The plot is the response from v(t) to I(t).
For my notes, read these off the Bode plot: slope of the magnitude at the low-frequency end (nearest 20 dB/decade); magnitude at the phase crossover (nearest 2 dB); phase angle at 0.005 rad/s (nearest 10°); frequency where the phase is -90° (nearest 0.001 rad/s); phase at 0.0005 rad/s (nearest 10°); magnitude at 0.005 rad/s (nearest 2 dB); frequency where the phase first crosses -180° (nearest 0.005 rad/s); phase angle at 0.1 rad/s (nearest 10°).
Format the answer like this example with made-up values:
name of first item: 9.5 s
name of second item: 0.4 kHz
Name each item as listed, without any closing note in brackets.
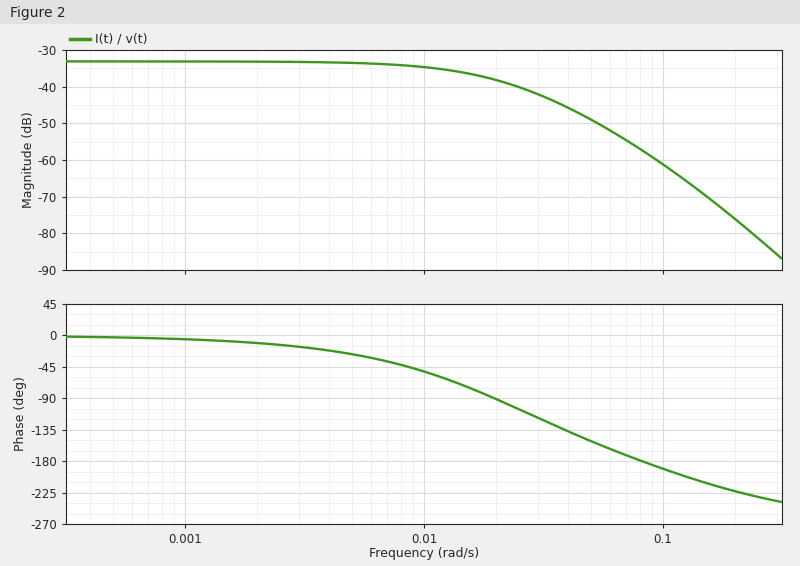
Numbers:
slope of the magnitude at the low-frequency end: 0 dB/decade
magnitude at the phase crossover: -58 dB
phase angle at 0.005 rad/s: -30°
frequency where the phase is -90°: 0.020 rad/s
phase at 0.0005 rad/s: 0°
magnitude at 0.005 rad/s: -34 dB
frequency where the phase first crosses -180°: 0.080 rad/s
phase angle at 0.1 rad/s: -190°
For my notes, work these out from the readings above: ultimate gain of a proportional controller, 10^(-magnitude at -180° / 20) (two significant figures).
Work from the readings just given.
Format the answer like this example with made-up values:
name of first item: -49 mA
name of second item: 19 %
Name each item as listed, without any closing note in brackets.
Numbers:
ultimate gain of a proportional controller, 10^(-magnitude at -180° / 20): 790
